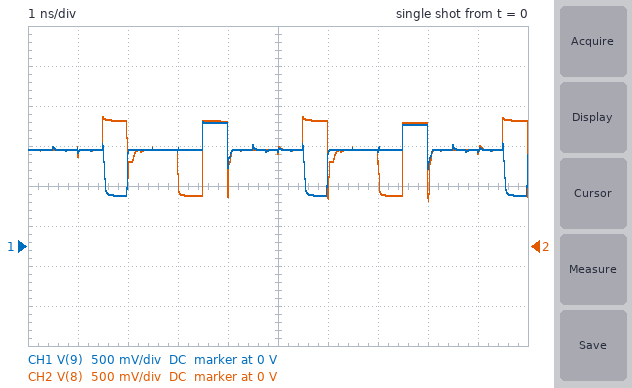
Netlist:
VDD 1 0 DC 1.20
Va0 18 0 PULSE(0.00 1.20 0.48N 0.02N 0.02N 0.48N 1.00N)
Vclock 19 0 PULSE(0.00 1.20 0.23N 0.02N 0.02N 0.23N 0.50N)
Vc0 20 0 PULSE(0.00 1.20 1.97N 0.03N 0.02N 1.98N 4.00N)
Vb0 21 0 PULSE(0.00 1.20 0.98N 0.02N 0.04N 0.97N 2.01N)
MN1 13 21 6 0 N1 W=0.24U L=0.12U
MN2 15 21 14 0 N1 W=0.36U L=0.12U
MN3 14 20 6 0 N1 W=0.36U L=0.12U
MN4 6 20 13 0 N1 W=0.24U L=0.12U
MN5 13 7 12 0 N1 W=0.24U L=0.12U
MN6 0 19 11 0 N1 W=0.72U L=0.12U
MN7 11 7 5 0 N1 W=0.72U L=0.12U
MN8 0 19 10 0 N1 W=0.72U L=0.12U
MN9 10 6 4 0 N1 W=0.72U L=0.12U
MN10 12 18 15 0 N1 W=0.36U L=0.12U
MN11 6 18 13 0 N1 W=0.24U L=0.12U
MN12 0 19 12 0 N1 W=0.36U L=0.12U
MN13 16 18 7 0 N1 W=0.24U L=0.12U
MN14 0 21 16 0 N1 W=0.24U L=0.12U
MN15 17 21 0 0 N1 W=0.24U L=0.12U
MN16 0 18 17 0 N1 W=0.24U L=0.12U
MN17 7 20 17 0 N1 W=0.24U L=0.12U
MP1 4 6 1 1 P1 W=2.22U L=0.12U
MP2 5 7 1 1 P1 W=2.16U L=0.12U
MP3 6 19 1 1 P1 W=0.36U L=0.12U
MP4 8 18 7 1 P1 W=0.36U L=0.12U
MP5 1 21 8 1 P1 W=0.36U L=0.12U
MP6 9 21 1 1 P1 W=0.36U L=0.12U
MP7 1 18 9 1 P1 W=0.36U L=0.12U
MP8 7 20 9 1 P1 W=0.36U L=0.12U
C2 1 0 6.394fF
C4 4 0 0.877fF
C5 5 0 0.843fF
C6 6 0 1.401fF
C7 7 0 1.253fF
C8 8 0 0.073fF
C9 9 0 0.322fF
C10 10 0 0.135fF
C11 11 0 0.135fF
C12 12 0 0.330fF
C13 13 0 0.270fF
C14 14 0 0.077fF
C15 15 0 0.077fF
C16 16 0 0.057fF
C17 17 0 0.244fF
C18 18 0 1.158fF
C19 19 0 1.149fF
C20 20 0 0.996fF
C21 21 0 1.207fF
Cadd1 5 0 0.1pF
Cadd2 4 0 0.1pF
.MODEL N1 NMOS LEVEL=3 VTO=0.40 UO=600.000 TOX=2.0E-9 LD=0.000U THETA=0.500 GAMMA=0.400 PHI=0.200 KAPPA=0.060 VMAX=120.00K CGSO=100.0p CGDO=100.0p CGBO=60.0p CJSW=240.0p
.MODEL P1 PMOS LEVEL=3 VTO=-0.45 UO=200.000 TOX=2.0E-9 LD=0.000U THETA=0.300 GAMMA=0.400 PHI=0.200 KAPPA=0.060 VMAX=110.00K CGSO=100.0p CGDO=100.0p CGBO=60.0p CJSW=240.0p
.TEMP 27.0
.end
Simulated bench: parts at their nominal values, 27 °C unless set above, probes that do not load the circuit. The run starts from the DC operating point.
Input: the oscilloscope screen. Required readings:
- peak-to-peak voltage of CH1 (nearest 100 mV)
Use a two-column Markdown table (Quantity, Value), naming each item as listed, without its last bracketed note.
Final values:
| Quantity | Value |
|---|---|
| peak-to-peak voltage of CH1 | 900 mV |
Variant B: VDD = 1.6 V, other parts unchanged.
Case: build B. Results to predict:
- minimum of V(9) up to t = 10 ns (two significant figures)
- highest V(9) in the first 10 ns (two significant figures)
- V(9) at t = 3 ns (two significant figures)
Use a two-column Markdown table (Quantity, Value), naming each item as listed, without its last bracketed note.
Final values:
| Quantity | Value |
|---|---|
| minimum of V(9) up to t = 10 ns | 700 mV |
| highest V(9) in the first 10 ns | 1.7 V |
| V(9) at t = 3 ns | 1.6 V |
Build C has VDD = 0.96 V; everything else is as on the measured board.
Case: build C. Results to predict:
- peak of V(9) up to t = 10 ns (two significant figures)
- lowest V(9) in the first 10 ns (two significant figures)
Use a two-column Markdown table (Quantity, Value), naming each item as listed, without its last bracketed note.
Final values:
| Quantity | Value |
|---|---|
| peak of V(9) up to t = 10 ns | 1.4 V |
| lowest V(9) in the first 10 ns | 580 mV |
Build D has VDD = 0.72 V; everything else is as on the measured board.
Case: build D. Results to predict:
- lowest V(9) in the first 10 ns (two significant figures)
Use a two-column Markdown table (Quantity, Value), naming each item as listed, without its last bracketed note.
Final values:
| Quantity | Value |
|---|---|
| lowest V(9) in the first 10 ns | 530 mV |
